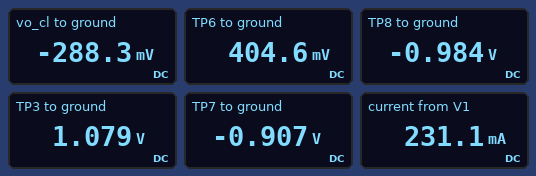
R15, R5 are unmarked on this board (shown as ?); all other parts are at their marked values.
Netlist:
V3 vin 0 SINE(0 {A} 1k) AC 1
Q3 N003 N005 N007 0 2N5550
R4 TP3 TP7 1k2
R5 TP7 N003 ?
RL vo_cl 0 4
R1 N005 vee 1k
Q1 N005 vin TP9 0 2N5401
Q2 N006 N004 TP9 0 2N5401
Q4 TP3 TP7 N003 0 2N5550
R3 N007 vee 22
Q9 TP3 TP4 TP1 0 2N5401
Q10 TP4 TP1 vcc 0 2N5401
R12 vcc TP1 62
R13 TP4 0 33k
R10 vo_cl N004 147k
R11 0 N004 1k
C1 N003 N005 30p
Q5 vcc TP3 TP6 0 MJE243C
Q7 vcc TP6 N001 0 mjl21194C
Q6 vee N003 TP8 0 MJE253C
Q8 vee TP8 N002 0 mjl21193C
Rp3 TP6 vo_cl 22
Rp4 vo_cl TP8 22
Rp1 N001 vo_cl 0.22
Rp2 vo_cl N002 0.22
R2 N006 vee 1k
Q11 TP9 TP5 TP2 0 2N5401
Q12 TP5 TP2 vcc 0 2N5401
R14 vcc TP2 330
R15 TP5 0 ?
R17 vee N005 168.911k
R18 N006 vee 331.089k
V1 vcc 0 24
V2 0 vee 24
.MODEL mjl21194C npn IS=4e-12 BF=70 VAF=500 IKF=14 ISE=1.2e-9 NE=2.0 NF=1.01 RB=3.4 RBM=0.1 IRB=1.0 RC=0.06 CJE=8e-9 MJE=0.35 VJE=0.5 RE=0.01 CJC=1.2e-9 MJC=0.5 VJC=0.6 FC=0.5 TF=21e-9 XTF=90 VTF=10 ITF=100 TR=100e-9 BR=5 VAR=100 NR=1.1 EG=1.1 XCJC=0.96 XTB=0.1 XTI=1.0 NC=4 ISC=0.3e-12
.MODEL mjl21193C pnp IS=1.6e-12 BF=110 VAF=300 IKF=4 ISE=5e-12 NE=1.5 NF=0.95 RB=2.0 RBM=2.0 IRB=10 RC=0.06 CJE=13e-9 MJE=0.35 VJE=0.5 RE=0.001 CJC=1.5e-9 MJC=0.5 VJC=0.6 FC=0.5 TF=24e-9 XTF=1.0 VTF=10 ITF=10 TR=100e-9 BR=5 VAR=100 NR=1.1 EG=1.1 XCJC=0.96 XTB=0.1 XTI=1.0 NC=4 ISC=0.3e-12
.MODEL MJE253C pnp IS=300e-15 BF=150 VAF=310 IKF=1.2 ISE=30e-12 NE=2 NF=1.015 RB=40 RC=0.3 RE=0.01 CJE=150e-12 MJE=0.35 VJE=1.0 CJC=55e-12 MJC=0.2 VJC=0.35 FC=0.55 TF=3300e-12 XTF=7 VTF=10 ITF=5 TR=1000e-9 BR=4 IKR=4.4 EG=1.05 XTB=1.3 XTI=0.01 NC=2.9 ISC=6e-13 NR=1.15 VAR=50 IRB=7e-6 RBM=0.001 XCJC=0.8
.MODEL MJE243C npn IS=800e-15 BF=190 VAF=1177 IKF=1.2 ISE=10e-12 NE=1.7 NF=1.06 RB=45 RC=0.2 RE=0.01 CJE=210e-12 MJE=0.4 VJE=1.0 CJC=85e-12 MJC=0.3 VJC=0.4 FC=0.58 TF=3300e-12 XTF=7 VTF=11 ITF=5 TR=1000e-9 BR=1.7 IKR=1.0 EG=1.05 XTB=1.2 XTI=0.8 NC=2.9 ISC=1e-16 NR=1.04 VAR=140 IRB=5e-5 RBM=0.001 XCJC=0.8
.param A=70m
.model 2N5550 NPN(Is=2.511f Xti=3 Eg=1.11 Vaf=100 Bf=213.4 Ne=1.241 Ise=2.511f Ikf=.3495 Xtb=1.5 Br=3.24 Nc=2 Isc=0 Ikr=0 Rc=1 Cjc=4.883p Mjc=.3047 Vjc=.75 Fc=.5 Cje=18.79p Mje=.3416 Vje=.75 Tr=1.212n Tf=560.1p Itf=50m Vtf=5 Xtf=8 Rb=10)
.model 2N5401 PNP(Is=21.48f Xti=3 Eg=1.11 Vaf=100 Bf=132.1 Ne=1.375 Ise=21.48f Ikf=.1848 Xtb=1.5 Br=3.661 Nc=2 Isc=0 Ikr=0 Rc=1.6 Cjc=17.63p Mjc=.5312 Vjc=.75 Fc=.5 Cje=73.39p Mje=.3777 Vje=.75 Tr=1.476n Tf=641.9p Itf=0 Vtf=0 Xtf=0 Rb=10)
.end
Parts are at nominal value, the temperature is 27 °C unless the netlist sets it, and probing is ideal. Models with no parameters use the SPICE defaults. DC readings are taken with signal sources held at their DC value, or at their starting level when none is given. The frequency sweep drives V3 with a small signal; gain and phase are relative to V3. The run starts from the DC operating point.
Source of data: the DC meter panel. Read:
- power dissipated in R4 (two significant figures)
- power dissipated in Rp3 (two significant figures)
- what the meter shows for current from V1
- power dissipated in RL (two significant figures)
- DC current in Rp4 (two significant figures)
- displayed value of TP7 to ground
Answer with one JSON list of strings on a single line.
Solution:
["3.3 mW", "22 mW", "231.1 mA", "21 mW", "32 mA", "-0.907 V"]
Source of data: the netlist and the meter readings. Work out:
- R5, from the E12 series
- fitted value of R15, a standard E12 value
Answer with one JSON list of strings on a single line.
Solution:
["470 Ω", "18 kΩ"]
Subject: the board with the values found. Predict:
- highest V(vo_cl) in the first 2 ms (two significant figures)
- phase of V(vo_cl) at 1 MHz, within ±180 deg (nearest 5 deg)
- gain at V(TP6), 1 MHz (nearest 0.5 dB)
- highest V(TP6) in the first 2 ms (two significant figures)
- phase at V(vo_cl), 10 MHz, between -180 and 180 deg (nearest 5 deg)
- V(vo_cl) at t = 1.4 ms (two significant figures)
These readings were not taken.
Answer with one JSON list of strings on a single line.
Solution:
["9.8 V", "-120 deg", "37.5 dB", "11 V", "130 deg", "5.7 V"]
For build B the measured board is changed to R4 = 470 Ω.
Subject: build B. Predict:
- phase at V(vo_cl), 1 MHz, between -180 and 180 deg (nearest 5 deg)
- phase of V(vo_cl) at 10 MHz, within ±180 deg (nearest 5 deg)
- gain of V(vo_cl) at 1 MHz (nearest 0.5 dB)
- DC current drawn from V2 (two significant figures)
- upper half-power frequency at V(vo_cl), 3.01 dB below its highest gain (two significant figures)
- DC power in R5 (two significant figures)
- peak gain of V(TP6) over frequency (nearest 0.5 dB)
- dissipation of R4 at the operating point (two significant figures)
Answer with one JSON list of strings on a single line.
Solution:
["-130 deg", "145 deg", "34.0 dB", "71 mA", "550 kHz", "1.2 mW", "43.0 dB", "1.3 mW"]
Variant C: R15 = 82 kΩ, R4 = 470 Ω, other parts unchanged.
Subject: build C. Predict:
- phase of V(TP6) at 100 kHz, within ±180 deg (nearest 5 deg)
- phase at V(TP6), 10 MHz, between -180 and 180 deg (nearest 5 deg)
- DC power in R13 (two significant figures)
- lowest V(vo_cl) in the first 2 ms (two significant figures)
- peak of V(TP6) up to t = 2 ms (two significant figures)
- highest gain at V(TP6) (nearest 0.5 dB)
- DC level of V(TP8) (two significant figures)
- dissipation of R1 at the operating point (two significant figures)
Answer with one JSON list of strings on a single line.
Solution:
["-15 deg", "110 deg", "16 mW", "-9.6 V", "12 V", "44.5 dB", "380 mV", "930 µW"]
